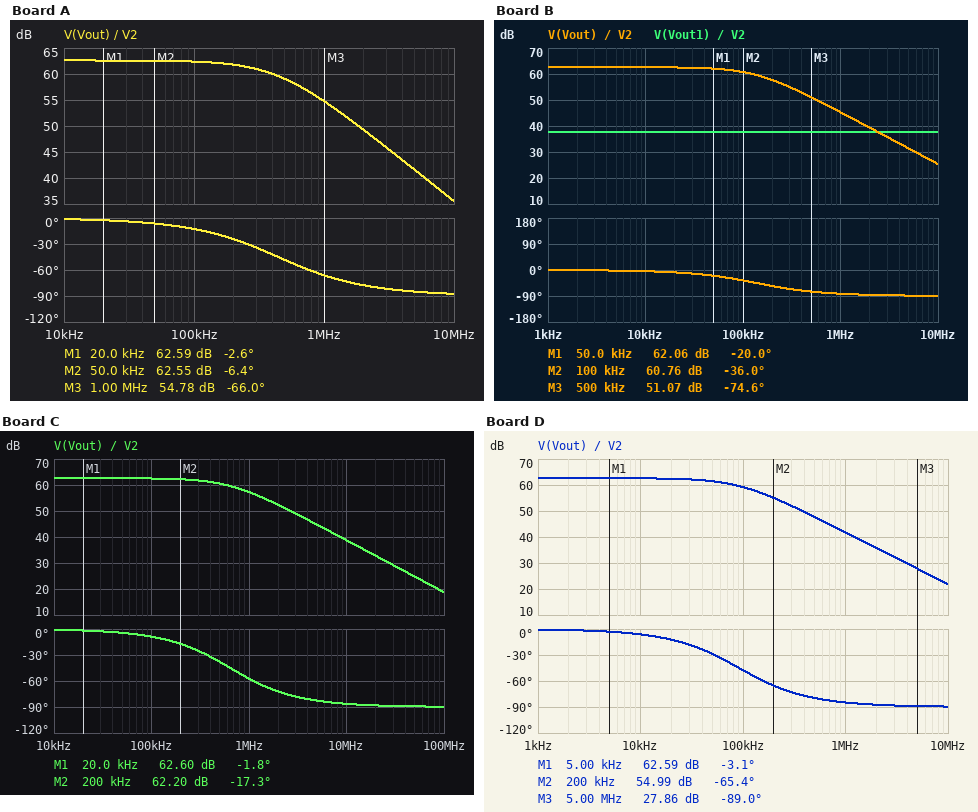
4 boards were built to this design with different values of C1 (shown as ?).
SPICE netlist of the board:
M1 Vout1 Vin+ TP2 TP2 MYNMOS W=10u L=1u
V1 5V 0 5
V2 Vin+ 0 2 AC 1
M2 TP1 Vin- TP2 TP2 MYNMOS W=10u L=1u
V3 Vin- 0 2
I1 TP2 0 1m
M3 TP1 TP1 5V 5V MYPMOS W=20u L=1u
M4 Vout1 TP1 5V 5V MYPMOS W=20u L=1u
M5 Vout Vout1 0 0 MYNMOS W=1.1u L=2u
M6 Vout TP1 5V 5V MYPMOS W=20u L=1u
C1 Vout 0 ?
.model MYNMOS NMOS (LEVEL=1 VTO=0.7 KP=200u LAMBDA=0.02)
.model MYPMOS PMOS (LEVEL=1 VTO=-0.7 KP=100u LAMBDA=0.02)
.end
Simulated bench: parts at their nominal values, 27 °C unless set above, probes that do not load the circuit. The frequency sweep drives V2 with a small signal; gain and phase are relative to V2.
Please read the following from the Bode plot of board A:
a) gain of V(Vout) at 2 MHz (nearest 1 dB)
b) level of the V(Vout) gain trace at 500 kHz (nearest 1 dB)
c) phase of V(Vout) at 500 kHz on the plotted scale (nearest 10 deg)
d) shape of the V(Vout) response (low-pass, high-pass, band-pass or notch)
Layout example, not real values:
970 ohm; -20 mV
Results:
49 dB; 59 dB; -50 deg; low-pass
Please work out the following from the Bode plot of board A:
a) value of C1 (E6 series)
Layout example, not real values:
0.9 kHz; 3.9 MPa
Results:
6.8 pF
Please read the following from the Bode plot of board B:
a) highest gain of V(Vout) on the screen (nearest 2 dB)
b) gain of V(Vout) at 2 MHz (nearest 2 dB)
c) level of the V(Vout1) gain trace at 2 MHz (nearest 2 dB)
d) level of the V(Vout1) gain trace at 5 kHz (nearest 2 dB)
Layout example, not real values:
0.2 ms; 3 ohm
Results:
62 dB; 40 dB; 38 dB; 38 dB
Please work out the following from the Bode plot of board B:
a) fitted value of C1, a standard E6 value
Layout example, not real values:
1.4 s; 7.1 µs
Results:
22 pF
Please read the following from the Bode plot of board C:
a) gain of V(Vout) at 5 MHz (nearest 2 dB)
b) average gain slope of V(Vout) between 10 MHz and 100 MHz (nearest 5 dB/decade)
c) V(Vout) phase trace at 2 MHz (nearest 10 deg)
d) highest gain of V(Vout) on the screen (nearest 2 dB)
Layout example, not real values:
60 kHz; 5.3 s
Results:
44 dB; -20 dB/decade; -70 deg; 62 dB
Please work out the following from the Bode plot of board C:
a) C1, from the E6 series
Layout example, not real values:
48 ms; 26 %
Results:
4.7 pF
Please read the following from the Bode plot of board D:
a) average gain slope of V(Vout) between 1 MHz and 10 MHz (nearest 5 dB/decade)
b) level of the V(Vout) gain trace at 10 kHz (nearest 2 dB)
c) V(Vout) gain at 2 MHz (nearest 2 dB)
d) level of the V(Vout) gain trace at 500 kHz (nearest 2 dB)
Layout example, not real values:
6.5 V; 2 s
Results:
-20 dB/decade; 62 dB; 36 dB; 48 dB
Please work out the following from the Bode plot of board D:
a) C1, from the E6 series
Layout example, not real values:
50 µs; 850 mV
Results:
33 pF
